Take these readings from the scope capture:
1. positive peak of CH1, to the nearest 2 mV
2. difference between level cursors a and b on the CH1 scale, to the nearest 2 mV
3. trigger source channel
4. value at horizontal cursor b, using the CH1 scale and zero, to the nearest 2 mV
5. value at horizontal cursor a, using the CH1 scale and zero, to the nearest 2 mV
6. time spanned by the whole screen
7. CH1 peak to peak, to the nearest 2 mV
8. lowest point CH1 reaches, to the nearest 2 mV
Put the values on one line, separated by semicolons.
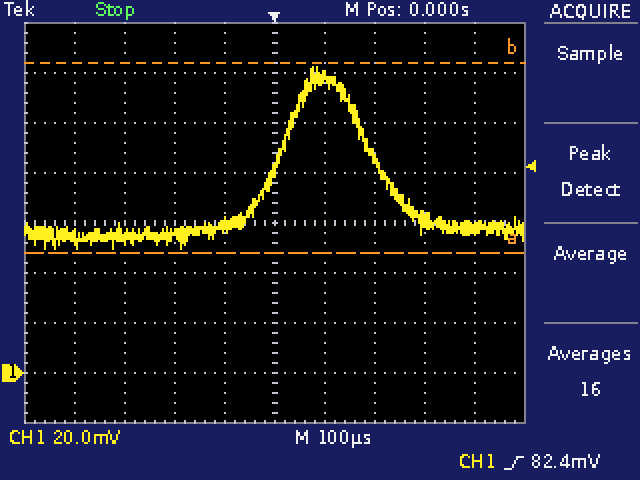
122 mV; 76 mV; CH1; 124 mV; 48 mV; 1 ms; 72 mV; 50 mV
